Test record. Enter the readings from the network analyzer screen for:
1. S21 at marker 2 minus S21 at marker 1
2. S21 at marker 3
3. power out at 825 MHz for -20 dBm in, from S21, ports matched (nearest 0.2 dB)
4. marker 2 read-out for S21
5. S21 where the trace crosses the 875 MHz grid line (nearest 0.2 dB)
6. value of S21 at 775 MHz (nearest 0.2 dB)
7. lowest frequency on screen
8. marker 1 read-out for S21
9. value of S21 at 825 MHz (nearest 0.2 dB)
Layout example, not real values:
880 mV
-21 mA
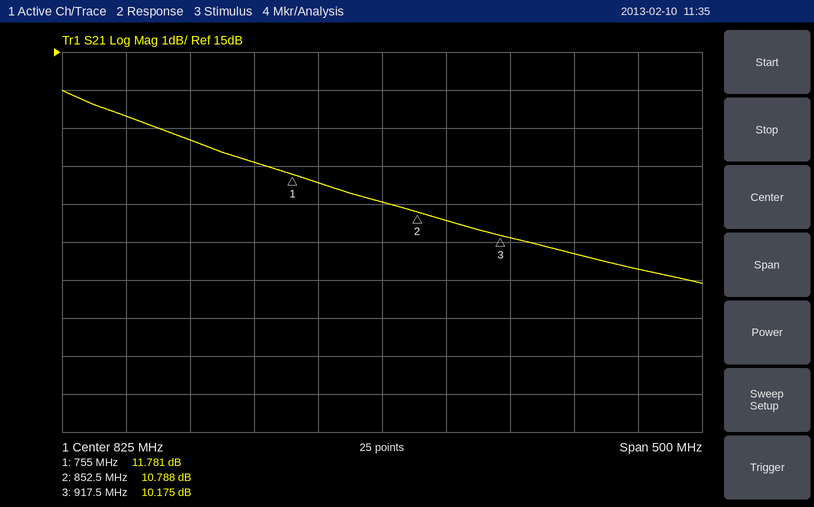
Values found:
-0.993 dB
10.175 dB
-9.0 dBm
10.788 dB
10.6 dB
11.6 dB
575 MHz
11.781 dB
11.0 dB
